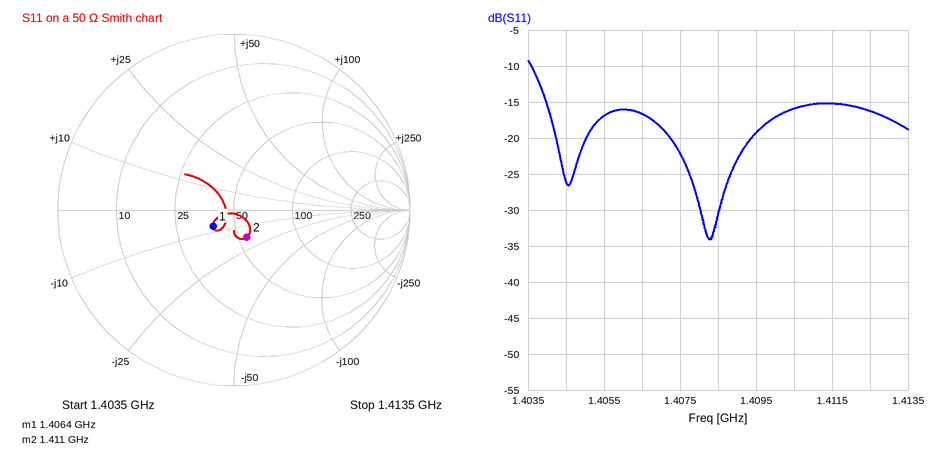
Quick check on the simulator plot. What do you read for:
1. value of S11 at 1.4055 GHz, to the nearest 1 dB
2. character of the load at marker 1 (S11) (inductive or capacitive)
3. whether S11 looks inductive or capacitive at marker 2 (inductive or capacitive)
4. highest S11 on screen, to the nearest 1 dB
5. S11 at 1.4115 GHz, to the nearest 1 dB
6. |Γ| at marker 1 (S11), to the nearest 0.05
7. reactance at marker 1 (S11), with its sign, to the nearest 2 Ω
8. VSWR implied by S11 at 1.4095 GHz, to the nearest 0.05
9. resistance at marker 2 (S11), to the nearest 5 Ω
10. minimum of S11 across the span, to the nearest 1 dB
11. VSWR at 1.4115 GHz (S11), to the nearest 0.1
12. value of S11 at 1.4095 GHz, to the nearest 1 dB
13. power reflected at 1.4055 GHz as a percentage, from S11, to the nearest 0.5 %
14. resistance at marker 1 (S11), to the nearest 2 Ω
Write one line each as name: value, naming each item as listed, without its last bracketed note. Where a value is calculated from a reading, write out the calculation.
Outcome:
value of S11 at 1.4055 GHz, to the nearest 1 dB: -17 dB
character of the load at marker 1 (S11): capacitive
whether S11 looks inductive or capacitive at marker 2: capacitive
highest S11 on screen, to the nearest 1 dB: -9 dB
S11 at 1.4115 GHz, to the nearest 1 dB: -15 dB
|Γ| at marker 1 (S11), to the nearest 0.05: 0.15
reactance at marker 1 (S11), with its sign, to the nearest 2 Ω: -8 Ω
VSWR implied by S11 at 1.4095 GHz, to the nearest 0.05: |Γ| = 10^(-19/20) = 0.1122; VSWR = (1 + 0.1122)/(1 − 0.1122) ≈ 1.25
resistance at marker 2 (S11), to the nearest 5 Ω: 55 Ω
minimum of S11 across the span, to the nearest 1 dB: -34 dB
VSWR at 1.4115 GHz (S11), to the nearest 0.1: |Γ| = 10^(-15/20) = 0.1778; VSWR = (1 + 0.1778)/(1 − 0.1778) ≈ 1.4
value of S11 at 1.4095 GHz, to the nearest 1 dB: -19 dB
power reflected at 1.4055 GHz as a percentage, from S11, to the nearest 0.5 %: 10^(-17/10) ≈ 2.0 %
resistance at marker 1 (S11), to the nearest 2 Ω: 38 Ω
